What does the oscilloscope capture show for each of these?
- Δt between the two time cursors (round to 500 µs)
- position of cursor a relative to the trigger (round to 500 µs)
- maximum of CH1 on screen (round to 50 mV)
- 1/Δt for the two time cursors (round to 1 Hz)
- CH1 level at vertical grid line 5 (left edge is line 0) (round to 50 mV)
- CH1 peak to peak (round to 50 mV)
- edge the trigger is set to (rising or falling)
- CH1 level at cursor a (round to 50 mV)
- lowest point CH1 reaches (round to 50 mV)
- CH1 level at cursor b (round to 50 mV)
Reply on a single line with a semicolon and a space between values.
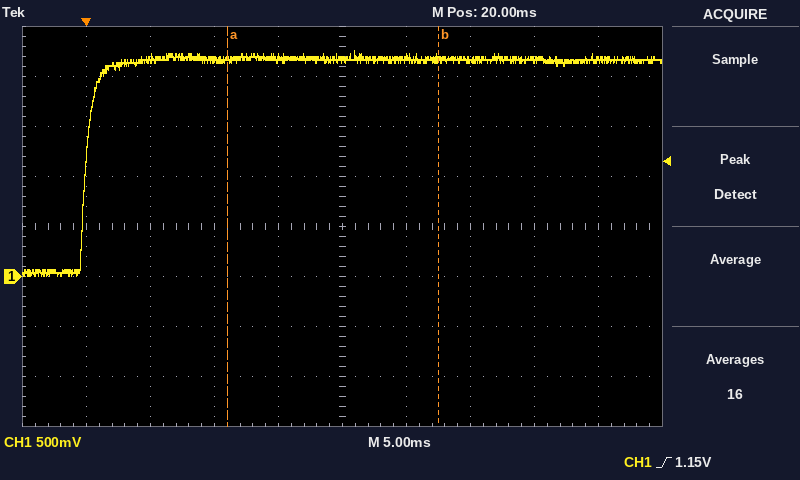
16.5 ms; +11.0 ms; 2.25 V; 61 Hz; 2.15 V; 2.25 V; rising; 2.15 V; 0 mV; 2.20 V
